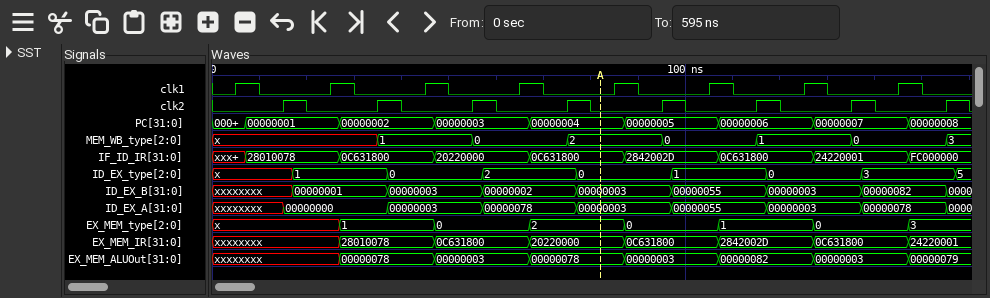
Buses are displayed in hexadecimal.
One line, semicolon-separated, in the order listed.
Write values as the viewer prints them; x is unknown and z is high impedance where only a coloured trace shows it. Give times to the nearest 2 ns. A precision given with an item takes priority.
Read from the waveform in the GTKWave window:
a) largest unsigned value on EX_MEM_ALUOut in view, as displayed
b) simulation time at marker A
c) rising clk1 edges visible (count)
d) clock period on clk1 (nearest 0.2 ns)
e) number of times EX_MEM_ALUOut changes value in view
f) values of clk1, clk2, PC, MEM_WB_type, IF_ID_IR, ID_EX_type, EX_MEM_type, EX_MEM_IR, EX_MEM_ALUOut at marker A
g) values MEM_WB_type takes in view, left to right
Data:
00000082; 82 ns; 8; 20 ns; 7; clk1=0, clk2=0, PC=00000004, MEM_WB_type=2, IF_ID_IR=0C631800, ID_EX_type=0, EX_MEM_type=2, EX_MEM_IR=20220000, EX_MEM_ALUOut=00000078; x, 1, 0, 2, 0, 1, 0, 3
